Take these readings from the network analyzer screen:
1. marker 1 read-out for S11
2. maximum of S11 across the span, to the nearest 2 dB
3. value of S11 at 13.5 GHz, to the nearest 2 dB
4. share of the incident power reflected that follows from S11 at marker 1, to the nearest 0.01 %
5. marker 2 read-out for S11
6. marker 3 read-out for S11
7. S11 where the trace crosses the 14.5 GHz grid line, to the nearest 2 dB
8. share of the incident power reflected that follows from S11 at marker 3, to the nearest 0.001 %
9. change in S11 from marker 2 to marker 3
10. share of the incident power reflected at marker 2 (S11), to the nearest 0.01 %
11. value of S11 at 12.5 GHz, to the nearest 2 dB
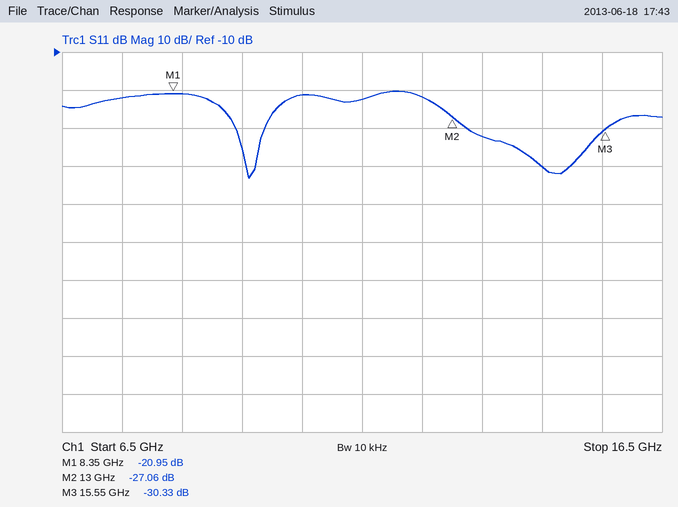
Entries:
-20.95 dB
-20 dB
-32 dB
0.80 %
-27.06 dB
-30.33 dB
-40 dB
0.093 %
-3.27 dB
0.20 %
-22 dB
